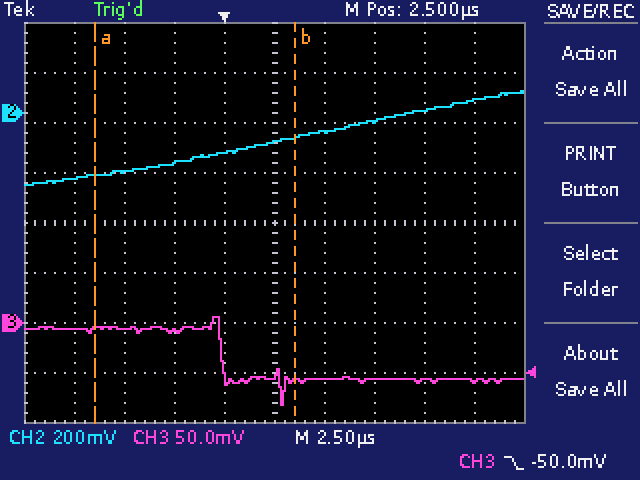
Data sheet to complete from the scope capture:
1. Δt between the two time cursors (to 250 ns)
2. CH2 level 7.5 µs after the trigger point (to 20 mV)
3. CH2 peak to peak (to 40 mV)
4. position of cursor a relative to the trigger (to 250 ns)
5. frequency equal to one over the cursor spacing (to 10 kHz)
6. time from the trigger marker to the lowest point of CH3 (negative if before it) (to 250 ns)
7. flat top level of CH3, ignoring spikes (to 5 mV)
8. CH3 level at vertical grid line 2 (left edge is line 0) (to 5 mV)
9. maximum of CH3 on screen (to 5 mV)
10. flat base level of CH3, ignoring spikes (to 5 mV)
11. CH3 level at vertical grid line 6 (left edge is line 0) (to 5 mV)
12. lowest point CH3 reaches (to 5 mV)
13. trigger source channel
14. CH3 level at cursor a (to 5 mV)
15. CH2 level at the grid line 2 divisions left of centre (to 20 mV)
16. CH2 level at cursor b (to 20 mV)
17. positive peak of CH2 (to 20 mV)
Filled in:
10.00 µs
-40 mV
360 mV
-6.50 µs
100 kHz
+3.00 µs
-5 mV
-5 mV
5 mV
-55 mV
-55 mV
-80 mV
CH3
-5 mV
-200 mV
-100 mV
80 mV
